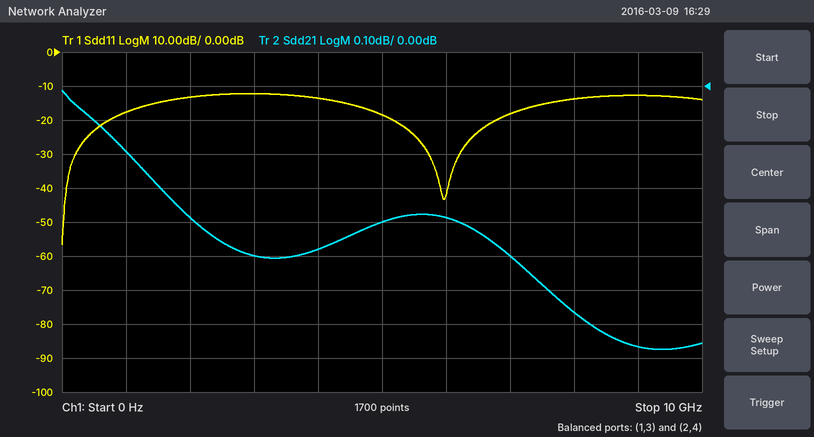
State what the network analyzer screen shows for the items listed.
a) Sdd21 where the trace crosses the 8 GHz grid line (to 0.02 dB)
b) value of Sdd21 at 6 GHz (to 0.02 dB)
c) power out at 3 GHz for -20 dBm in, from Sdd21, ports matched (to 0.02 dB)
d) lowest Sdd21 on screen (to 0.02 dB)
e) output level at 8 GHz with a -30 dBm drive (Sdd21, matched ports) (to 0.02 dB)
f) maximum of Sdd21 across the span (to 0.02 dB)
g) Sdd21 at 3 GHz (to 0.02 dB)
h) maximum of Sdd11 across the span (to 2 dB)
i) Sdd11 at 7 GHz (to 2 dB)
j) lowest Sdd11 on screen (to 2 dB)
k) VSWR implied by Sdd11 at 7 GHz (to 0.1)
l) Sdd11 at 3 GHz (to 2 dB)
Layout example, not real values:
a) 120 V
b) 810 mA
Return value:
a) -0.66 dB
b) -0.38 dB
c) -20.50 dBm
d) -0.78 dB
e) -30.66 dBm
f) -0.02 dB
g) -0.50 dB
h) -12 dB
i) -18 dB
j) -56 dB
k) 1.3
l) -12 dB
